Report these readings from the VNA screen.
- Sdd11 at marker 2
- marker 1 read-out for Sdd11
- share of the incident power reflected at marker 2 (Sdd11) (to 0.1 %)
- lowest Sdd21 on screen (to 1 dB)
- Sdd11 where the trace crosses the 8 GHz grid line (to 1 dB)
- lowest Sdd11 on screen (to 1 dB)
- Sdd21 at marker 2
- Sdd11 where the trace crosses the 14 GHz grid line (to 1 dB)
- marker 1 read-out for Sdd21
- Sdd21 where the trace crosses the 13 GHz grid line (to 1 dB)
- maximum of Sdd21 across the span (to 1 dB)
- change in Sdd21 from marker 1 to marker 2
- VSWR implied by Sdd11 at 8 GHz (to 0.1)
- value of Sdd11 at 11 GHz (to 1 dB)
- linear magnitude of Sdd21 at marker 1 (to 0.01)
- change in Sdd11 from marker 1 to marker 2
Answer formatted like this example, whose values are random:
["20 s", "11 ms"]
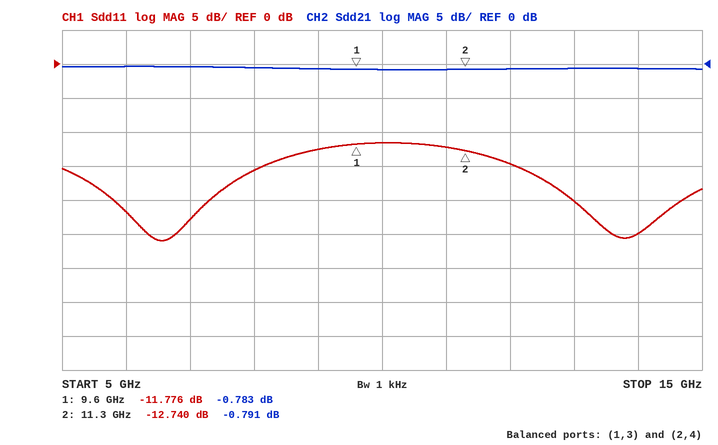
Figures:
["-12.740 dB", "-11.776 dB", "5.3 %", "-1 dB", "-16 dB", "-26 dB", "-0.791 dB", "-25 dB", "-0.783 dB", "-1 dB", "0 dB", "-0.008 dB", "1.4", "-12 dB", "0.91", "-0.964 dB"]
